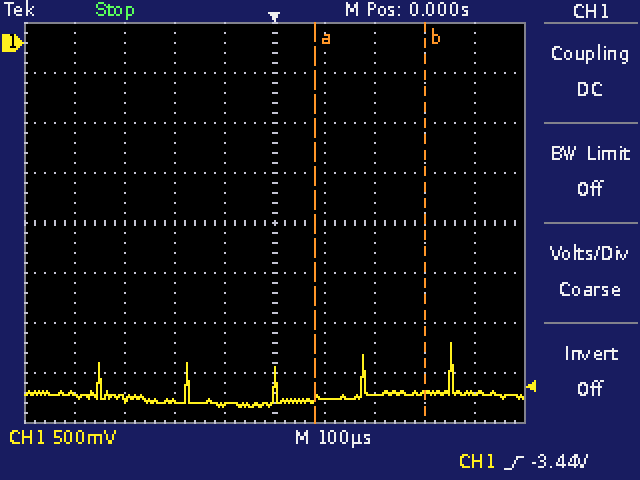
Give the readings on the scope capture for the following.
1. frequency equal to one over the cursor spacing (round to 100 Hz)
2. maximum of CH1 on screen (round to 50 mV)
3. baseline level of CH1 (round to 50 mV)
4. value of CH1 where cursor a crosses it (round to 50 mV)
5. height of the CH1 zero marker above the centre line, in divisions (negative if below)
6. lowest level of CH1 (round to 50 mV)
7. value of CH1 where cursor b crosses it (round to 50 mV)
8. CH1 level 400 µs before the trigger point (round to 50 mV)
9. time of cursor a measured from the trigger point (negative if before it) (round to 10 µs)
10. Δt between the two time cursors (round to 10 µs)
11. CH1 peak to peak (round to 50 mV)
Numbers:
4.5 kHz
-3.00 V
-3.50 V
-3.55 V
+3.6 div
-3.65 V
-3.50 V
-3.50 V
+80 µs
220 µs
650 mV
